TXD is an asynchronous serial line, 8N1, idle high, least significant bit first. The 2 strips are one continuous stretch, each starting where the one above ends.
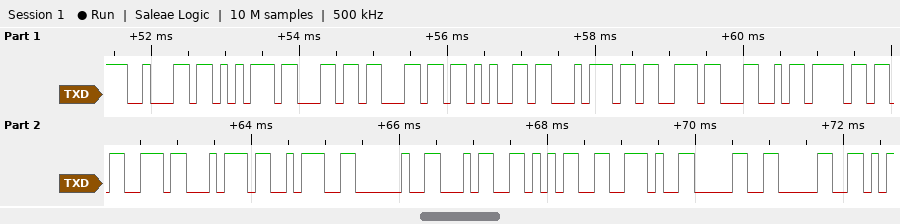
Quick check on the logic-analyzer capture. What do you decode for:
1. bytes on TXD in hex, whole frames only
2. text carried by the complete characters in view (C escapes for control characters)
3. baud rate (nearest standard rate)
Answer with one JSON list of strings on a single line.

["62 75 6C 6C 65 74 73 4C 6F 73 74 3A 20 34 35 2E 30 30", "\"bulletsLost: 45.00\"", "9600 baud"]
